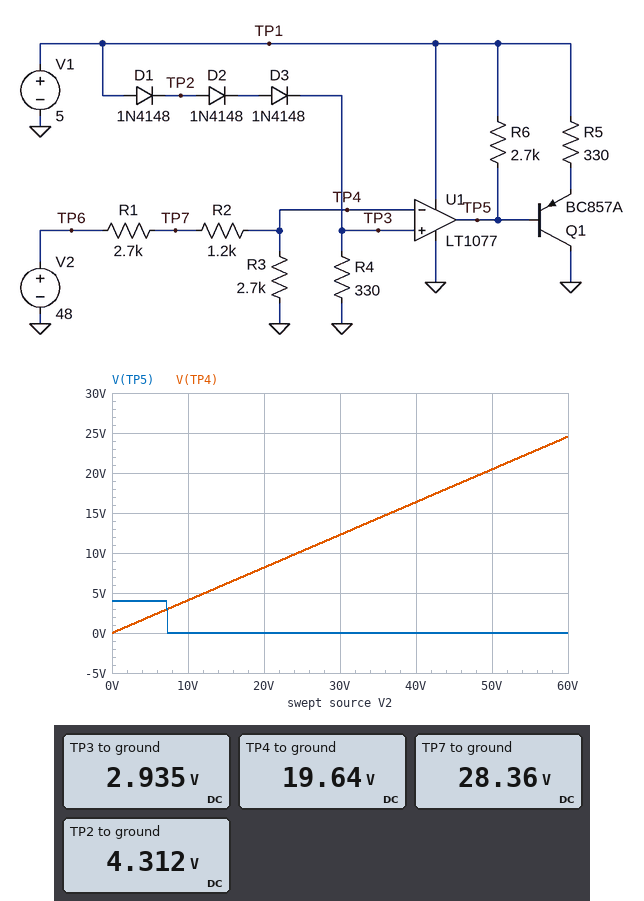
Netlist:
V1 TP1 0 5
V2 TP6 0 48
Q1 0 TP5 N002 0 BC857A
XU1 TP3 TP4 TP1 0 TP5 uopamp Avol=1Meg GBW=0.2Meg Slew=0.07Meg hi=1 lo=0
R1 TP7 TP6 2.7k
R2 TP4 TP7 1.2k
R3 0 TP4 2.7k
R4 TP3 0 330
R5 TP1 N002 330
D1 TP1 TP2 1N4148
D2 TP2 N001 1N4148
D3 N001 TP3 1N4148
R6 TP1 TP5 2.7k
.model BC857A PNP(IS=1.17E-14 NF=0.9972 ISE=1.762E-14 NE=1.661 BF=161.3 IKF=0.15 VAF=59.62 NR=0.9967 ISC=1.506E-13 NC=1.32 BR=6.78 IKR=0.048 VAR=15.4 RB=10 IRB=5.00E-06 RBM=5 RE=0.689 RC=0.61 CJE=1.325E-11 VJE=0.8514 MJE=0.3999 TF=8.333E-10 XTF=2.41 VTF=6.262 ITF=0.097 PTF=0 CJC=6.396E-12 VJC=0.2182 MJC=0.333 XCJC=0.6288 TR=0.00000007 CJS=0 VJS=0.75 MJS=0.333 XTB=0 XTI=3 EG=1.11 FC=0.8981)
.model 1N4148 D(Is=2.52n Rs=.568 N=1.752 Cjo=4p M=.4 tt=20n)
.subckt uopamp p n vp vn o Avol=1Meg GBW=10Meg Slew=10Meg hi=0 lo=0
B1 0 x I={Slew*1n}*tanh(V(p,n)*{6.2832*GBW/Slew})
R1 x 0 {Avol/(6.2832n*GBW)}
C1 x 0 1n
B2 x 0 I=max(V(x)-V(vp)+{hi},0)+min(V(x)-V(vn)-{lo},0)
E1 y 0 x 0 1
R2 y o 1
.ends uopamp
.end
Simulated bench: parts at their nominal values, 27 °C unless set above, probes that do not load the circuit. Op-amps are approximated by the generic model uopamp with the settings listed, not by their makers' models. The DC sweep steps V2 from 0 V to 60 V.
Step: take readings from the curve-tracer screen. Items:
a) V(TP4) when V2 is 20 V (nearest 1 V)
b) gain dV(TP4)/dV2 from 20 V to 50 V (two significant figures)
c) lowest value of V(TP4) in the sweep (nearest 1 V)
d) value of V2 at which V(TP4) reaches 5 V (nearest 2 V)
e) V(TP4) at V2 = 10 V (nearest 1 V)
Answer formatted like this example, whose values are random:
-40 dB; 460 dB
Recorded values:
8 V; 0.41 V/V; 0 V; 12 V; 4 V
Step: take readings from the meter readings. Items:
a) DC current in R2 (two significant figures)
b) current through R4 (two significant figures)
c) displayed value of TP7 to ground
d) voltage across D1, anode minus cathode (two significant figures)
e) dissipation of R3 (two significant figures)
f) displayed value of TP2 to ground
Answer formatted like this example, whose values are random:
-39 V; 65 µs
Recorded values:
7.3 mA; 8.9 mA; 28.36 V; 690 mV; 140 mW; 4.312 V
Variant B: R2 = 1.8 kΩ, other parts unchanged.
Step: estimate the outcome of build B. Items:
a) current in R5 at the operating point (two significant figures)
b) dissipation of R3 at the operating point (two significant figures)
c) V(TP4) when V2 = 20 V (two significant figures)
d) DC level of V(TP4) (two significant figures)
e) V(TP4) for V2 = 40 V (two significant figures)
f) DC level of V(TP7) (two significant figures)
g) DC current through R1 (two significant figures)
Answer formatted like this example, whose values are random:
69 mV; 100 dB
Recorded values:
13 mA; 120 mW; 7.5 V; 18 V; 15 V; 30 V; 6.7 mA
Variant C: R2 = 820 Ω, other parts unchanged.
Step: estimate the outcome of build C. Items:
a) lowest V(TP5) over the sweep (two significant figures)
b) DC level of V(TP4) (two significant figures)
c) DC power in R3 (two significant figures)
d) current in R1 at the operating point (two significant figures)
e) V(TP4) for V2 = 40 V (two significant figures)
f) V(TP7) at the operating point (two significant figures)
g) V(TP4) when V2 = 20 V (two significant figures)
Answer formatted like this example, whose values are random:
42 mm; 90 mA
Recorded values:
1.9 mV; 21 V; 160 mW; 7.7 mA; 17 V; 27 V; 8.7 V
